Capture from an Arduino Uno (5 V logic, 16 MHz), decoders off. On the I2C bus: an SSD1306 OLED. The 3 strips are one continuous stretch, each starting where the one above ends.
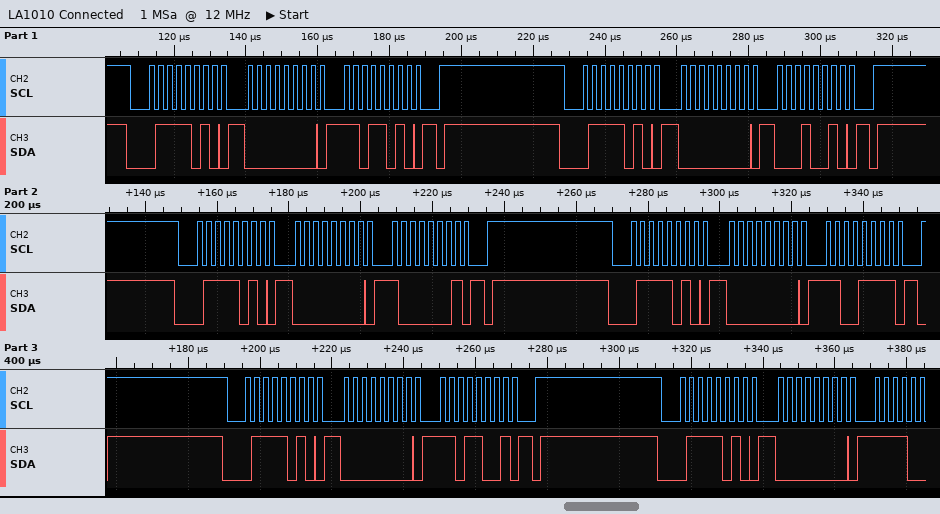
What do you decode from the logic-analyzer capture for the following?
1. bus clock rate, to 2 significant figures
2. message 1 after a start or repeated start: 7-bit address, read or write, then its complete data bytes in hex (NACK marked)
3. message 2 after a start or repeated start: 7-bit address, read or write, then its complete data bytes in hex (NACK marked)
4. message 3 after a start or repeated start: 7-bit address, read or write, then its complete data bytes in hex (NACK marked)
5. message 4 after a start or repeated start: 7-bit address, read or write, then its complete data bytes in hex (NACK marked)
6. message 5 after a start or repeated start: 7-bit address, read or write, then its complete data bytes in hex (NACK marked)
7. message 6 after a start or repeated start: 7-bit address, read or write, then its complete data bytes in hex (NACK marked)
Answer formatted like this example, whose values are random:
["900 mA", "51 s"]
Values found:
["400 kHz", "0x3D write: 00 DA", "0x3D write: 00 12", "0x3D write: 00 81", "0x3D write: 00 CF", "0x3D write: 00 D9", "0x3D write: 00"]
